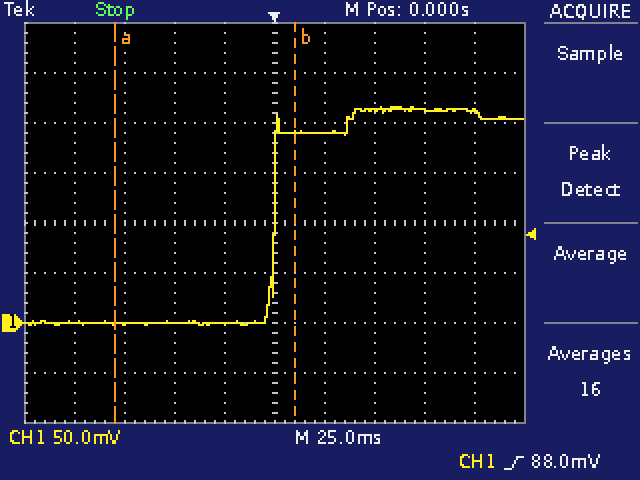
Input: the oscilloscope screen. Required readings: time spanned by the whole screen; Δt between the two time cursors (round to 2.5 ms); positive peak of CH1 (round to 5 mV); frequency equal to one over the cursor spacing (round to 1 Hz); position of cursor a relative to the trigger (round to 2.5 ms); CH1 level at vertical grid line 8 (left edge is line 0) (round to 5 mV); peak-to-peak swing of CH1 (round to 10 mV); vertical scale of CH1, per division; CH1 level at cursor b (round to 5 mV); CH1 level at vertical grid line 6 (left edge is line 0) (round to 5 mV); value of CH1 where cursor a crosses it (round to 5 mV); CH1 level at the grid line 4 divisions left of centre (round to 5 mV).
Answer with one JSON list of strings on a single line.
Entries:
["250 ms", "90.0 ms", "215 mV", "11 Hz", "-80.0 ms", "215 mV", "220 mV", "50 mV", "190 mV", "190 mV", "0 mV", "0 mV"]
